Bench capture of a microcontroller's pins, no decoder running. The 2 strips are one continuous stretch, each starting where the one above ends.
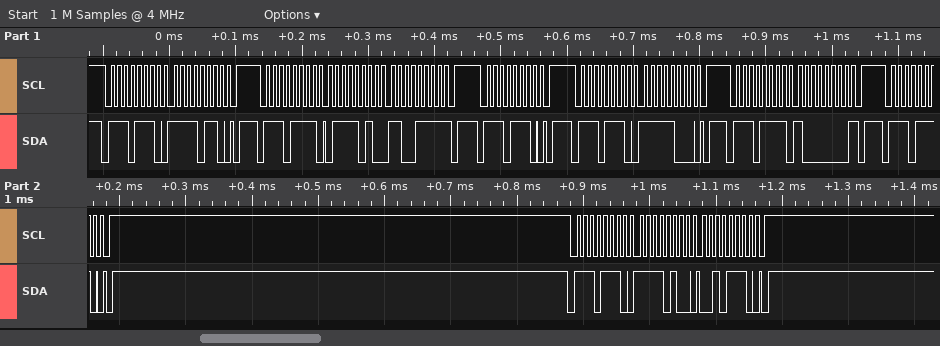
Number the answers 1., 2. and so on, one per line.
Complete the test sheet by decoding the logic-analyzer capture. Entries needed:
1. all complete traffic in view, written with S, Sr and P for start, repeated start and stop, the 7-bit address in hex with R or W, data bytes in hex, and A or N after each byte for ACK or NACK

1. S 77W A F6 A P S 77R A 7A A CF N P S 77W A P S 77W A F8 A P S 77R A 80 N P S 77W A P S 77W A F4 A 2E A P
